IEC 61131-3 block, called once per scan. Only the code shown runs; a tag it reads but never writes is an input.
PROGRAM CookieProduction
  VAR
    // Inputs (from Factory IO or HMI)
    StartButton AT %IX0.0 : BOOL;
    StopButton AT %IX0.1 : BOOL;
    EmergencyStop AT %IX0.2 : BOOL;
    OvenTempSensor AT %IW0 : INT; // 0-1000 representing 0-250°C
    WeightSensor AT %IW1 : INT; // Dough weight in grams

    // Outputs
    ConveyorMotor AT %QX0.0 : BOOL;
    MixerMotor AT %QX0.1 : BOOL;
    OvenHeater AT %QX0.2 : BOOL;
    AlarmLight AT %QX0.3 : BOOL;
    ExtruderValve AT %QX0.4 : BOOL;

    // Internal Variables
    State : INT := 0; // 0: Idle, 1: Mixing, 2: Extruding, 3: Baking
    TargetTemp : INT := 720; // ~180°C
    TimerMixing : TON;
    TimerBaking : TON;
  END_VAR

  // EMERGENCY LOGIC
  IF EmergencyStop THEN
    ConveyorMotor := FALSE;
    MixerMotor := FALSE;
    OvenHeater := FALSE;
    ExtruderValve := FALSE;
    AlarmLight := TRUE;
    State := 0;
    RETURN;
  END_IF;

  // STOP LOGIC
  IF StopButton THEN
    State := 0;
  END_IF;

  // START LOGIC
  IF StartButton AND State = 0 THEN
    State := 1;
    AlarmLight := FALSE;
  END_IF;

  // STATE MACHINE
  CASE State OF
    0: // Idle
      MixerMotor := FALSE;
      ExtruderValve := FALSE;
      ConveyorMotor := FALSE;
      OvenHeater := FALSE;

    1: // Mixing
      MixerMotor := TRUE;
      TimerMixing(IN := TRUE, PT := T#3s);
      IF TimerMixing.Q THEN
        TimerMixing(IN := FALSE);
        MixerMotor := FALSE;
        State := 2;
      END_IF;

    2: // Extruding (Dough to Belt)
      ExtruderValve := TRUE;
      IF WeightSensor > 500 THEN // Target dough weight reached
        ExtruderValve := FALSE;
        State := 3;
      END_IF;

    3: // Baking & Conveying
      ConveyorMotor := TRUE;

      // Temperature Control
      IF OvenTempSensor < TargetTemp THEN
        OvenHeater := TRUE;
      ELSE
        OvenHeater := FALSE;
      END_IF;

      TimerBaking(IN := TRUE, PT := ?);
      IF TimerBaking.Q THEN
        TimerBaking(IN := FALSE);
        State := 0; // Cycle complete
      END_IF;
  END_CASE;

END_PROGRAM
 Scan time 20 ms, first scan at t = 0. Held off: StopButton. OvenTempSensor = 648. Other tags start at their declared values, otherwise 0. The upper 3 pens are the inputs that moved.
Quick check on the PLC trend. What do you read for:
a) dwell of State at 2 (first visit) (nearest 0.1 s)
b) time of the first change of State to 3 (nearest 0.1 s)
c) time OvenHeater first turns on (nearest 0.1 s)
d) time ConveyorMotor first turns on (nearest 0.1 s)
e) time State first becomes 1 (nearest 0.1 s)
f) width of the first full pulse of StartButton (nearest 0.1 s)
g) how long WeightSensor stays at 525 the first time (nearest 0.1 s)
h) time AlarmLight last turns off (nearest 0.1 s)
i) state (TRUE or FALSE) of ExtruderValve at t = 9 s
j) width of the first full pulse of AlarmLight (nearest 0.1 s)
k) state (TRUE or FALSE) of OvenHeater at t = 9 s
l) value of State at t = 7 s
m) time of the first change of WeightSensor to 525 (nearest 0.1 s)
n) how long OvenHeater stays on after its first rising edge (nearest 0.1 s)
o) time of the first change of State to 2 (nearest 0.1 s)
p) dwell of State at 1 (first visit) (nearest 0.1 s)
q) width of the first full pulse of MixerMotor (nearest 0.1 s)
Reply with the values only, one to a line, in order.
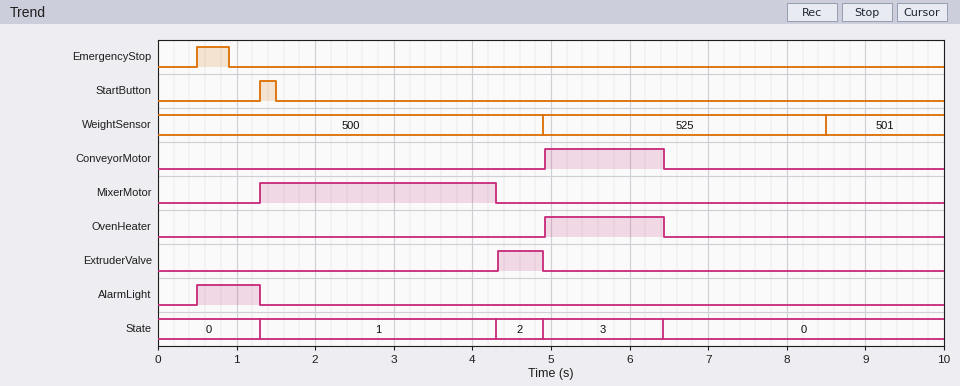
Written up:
0.6 s
4.9 s
4.9 s
4.9 s
1.3 s
0.2 s
3.6 s
1.3 s
FALSE
0.8 s
FALSE
0
4.9 s
1.5 s
4.3 s
3.0 s
3.0 s
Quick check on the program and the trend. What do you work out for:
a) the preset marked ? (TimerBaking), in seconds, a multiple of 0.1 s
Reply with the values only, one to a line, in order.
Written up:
1.5 s
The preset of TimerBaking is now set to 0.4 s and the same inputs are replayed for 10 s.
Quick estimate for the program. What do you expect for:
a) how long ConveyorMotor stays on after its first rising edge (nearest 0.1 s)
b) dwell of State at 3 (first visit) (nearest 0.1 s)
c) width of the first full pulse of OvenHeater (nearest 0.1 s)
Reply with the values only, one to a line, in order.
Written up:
0.4 s
0.4 s
0.4 s
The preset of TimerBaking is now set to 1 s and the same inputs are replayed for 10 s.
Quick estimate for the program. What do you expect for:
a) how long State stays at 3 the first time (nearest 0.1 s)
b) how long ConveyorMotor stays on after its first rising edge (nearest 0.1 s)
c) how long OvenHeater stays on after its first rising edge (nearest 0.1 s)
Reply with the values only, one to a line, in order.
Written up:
1.0 s
1.0 s
1.0 s
